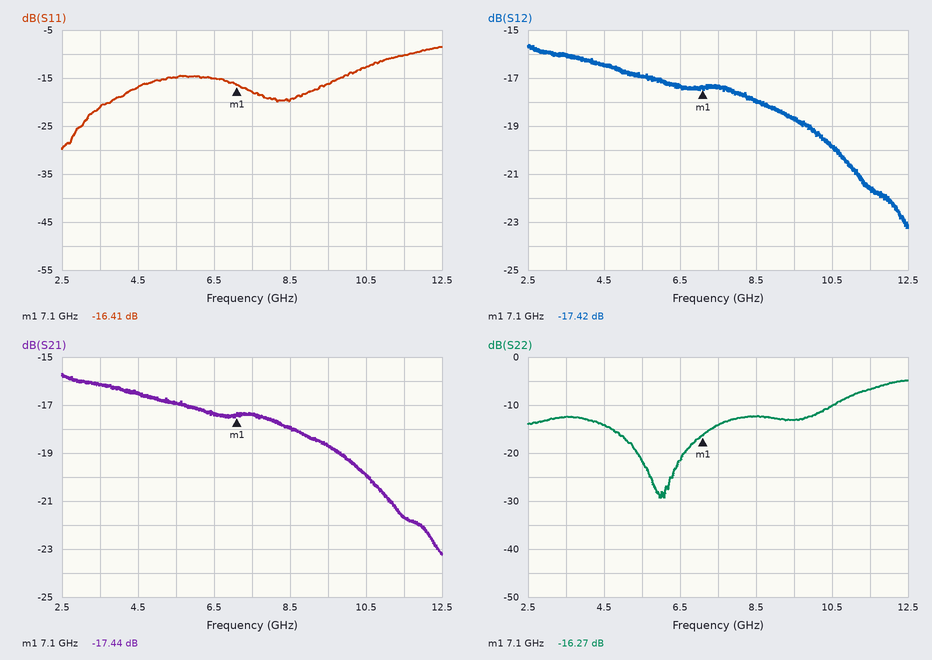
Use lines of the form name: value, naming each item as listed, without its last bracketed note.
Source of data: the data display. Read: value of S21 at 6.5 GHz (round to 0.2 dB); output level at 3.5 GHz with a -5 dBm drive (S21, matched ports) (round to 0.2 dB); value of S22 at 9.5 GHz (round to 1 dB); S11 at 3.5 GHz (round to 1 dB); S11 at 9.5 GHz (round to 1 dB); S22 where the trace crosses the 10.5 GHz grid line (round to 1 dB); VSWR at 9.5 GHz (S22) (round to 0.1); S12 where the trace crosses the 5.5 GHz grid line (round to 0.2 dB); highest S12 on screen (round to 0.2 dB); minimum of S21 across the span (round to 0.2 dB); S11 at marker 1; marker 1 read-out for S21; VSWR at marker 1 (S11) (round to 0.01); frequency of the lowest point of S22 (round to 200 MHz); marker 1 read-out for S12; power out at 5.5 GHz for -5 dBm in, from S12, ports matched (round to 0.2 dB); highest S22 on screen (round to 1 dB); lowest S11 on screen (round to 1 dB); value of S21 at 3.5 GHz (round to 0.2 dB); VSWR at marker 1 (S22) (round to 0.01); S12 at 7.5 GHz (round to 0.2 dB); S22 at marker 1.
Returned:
value of S21 at 6.5 GHz: -17.4 dB
output level at 3.5 GHz with a -5 dBm drive (S21, matched ports): -21.2 dBm
value of S22 at 9.5 GHz: -13 dB
S11 at 3.5 GHz: -21 dB
S11 at 9.5 GHz: -16 dB
S22 where the trace crosses the 10.5 GHz grid line: -10 dB
VSWR at 9.5 GHz (S22): 1.6
S12 where the trace crosses the 5.5 GHz grid line: -17.0 dB
highest S12 on screen: -15.6 dB
minimum of S21 across the span: -23.2 dB
S11 at marker 1: -16.41 dB
marker 1 read-out for S21: -17.44 dB
VSWR at marker 1 (S11): 1.36
frequency of the lowest point of S22: 6.0 GHz
marker 1 read-out for S12: -17.42 dB
power out at 5.5 GHz for -5 dBm in, from S12, ports matched: -22.0 dBm
highest S22 on screen: -5 dB
lowest S11 on screen: -30 dB
value of S21 at 3.5 GHz: -16.2 dB
VSWR at marker 1 (S22): 1.36
S12 at 7.5 GHz: -17.4 dB
S22 at marker 1: -16.27 dB
